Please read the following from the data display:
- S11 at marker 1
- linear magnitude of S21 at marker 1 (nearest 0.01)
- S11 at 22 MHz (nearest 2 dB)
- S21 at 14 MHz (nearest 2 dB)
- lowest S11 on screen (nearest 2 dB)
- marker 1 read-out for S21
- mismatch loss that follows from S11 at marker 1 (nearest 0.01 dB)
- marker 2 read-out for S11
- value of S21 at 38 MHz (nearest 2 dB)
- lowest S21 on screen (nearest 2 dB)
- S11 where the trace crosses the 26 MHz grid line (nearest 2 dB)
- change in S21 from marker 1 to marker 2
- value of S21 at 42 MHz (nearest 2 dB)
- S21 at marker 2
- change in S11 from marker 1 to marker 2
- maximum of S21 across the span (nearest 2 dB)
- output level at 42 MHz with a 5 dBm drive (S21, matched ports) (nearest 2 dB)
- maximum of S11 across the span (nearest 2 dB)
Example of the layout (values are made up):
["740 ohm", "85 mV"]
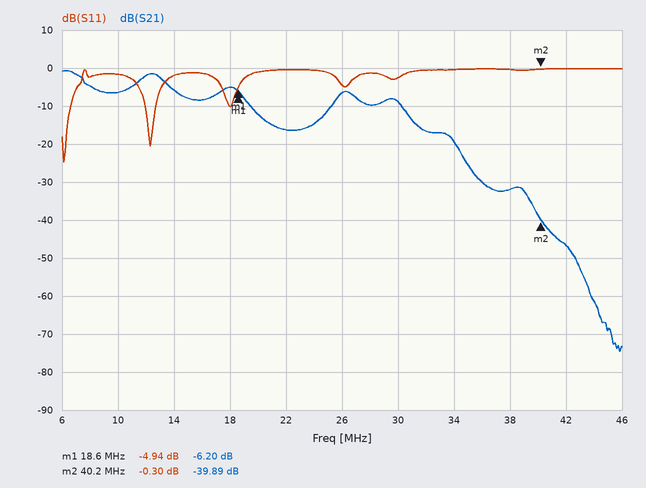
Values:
["-4.94 dB", "0.49", "0 dB", "-6 dB", "-24 dB", "-6.20 dB", "1.68 dB", "-0.30 dB", "-32 dB", "-74 dB", "-4 dB", "-33.69 dB", "-46 dB", "-39.89 dB", "4.64 dB", "0 dB", "-42 dBm", "0 dB"]
